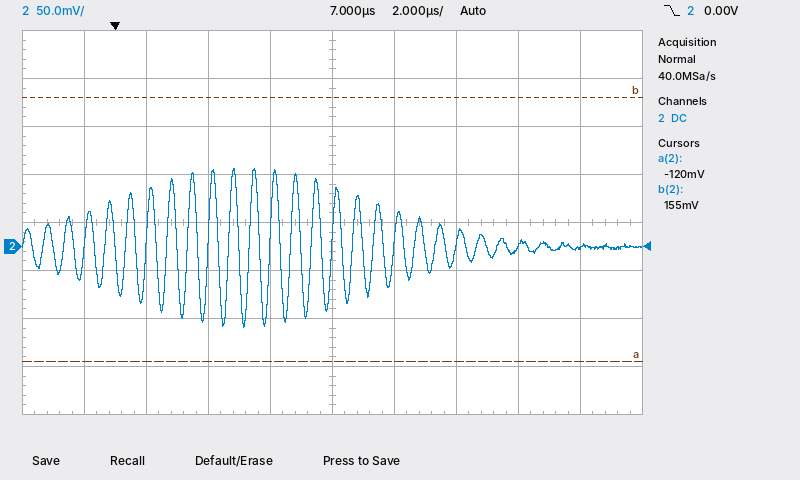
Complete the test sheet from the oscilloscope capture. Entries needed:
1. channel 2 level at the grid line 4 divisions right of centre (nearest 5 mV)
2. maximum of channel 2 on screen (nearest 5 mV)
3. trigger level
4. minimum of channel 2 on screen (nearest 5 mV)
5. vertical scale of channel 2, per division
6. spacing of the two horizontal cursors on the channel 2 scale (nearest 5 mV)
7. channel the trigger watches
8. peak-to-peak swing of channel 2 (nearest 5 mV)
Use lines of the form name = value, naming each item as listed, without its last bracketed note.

channel 2 level at the grid line 4 divisions right of centre = 0 mV
maximum of channel 2 on screen = 80 mV
trigger level = 0.00 V
minimum of channel 2 on screen = -85 mV
vertical scale of channel 2, per division = 50 mV
spacing of the two horizontal cursors on the channel 2 scale = 275 mV
channel the trigger watches = channel 2
peak-to-peak swing of channel 2 = 165 mV
